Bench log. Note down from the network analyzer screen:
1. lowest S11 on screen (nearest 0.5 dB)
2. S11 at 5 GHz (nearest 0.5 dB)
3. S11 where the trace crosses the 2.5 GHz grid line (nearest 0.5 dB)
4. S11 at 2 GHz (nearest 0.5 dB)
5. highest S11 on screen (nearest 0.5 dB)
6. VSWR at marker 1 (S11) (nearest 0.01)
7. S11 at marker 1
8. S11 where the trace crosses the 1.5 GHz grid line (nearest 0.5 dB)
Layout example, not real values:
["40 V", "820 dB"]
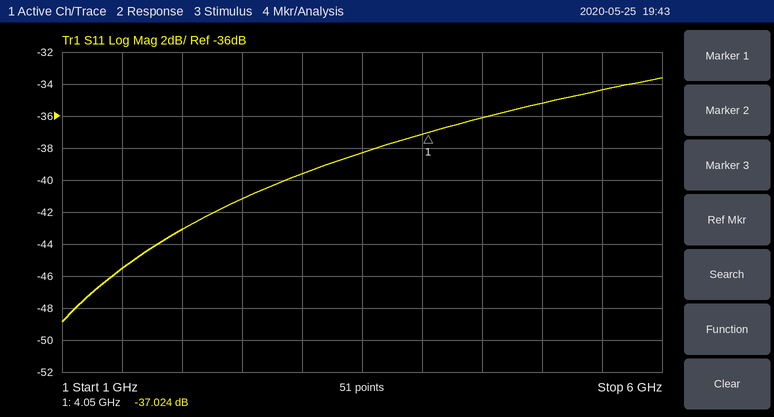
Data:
["-49.0 dB", "-35.0 dB", "-41.0 dB", "-43.0 dB", "-33.5 dB", "1.03", "-37.024 dB", "-45.5 dB"]
